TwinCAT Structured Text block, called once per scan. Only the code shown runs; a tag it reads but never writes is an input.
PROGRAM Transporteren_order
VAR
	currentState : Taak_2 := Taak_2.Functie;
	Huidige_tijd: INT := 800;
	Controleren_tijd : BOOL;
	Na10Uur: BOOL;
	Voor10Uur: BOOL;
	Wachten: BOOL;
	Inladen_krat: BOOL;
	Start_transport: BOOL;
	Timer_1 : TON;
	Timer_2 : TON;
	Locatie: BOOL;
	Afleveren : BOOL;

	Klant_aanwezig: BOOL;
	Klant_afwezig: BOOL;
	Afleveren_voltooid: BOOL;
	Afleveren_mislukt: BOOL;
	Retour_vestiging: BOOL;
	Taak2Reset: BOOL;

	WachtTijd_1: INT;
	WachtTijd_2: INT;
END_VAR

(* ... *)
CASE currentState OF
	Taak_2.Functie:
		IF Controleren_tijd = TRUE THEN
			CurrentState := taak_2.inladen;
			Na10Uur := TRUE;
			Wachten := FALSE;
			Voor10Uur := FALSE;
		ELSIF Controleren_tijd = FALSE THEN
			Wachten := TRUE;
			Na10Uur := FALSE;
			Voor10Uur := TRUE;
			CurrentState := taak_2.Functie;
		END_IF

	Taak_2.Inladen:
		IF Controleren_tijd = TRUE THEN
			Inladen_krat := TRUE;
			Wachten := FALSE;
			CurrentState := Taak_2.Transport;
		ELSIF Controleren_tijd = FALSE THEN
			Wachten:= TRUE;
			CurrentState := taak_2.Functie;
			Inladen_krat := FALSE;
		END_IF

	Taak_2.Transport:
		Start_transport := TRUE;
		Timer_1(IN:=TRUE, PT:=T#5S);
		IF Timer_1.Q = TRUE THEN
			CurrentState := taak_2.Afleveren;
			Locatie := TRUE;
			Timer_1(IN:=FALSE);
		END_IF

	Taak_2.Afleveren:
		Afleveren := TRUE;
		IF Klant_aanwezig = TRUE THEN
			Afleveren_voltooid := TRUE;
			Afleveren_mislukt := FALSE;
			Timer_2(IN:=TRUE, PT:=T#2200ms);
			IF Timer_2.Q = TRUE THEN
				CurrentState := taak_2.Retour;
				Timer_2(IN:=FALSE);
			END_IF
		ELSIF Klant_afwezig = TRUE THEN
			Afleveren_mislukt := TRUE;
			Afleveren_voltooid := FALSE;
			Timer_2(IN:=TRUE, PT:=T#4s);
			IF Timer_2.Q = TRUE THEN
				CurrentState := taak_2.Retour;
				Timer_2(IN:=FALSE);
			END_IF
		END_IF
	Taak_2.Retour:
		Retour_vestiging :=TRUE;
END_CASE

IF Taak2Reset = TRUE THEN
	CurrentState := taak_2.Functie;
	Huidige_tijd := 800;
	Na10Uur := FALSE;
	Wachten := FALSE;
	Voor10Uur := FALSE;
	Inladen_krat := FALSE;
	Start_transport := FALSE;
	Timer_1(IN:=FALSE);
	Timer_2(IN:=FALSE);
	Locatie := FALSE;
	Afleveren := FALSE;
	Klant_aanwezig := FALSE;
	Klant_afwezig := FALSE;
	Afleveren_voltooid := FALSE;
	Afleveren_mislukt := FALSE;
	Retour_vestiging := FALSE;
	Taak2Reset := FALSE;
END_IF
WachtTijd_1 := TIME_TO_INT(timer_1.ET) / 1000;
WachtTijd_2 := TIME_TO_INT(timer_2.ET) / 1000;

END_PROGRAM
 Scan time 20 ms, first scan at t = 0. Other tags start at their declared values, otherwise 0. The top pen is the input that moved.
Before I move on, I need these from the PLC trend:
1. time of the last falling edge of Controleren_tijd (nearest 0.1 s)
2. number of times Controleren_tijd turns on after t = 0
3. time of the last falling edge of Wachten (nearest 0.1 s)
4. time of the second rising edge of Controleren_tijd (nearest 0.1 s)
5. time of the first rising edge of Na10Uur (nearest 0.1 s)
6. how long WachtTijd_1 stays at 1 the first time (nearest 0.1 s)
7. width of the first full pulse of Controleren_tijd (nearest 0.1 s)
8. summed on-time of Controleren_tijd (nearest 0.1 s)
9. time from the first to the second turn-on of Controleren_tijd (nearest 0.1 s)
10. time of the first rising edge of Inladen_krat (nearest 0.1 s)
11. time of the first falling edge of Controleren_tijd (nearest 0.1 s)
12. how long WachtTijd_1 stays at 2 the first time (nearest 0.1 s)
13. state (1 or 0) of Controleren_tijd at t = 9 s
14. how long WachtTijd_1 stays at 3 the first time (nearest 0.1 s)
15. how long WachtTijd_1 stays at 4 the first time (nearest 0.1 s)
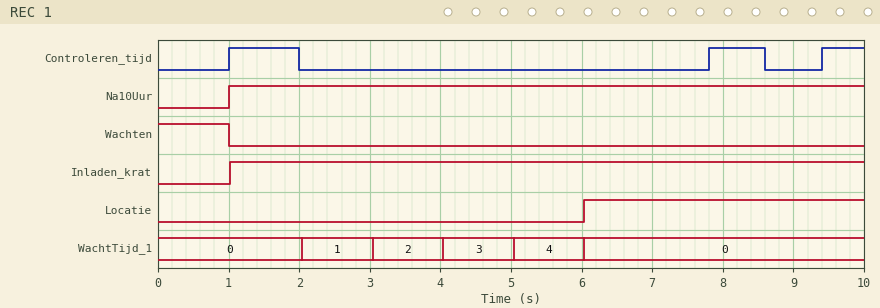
8.6 s
3
1.0 s
7.8 s
1.0 s
1.0 s
1.0 s
2.4 s
6.8 s
1.0 s
2.0 s
1.0 s
0
1.0 s
1.0 s
